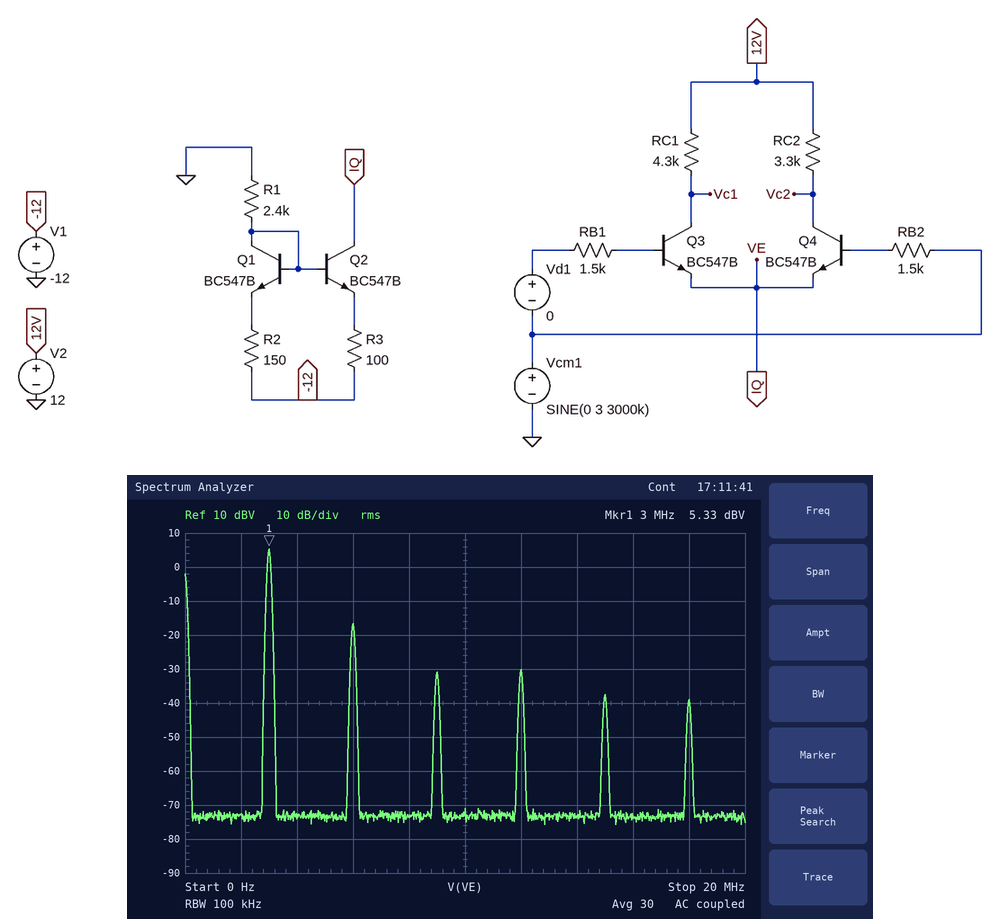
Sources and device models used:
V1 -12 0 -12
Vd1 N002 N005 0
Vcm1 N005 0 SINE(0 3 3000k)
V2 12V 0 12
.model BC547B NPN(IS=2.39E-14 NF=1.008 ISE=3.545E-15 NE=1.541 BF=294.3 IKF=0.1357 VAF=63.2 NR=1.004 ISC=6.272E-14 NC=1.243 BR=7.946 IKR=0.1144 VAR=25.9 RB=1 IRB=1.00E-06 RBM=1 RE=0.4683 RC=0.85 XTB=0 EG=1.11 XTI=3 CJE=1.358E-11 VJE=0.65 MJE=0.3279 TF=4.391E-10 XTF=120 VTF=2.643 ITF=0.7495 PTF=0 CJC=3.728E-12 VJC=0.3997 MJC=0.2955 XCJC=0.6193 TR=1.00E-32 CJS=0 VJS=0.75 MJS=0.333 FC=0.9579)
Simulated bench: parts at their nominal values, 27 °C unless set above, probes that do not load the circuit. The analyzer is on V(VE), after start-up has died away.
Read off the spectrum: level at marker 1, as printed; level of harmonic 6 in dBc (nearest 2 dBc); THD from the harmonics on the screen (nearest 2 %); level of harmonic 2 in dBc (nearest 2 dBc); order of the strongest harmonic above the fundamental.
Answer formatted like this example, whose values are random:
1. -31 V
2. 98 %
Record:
1. 5.33 dBV
2. -44 dBc
3. 8 %
4. -22 dBc
5. 2
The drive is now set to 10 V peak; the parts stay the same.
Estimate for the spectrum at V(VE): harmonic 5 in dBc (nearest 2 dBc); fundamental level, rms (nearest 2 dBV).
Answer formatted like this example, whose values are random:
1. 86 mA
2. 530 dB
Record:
1. -46 dBc
2. 16 dBV
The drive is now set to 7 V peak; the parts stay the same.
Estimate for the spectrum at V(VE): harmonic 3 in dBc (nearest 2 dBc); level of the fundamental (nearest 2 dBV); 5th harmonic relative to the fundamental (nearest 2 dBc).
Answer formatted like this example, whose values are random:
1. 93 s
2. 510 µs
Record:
1. -38 dBc
2. 12 dBV
3. -44 dBc
